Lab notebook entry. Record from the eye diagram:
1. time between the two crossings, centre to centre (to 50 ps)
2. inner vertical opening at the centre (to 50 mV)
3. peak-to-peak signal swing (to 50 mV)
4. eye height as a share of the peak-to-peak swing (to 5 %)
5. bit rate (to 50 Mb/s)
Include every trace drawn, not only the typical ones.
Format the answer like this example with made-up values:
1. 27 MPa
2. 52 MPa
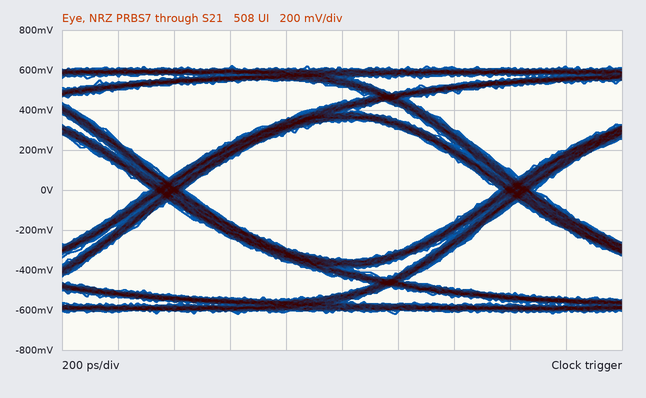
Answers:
1. 1.25 ns
2. 700 mV
3. 1.25 V
4. 55 %
5. 800 Mb/s
